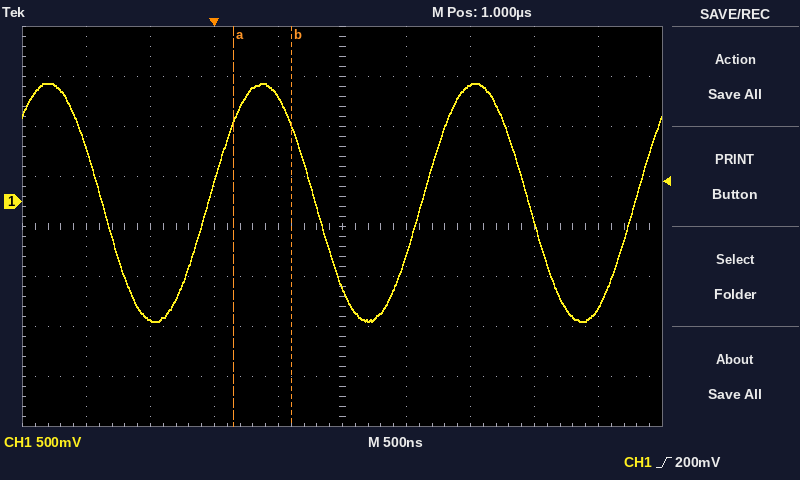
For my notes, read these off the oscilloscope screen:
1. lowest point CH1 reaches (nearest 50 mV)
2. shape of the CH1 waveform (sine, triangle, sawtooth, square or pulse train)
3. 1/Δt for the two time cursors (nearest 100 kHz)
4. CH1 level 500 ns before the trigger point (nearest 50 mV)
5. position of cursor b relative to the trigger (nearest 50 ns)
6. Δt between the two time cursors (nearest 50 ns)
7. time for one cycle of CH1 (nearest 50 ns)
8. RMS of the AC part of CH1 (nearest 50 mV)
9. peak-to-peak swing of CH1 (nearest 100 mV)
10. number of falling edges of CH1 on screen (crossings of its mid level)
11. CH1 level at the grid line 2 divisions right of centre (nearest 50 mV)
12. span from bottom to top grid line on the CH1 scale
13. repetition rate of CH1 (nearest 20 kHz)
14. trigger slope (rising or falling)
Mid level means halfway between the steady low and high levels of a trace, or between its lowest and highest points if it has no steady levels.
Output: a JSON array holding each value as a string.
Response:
["-1.20 V", "sine", "2.2 MHz", "-1.20 V", "+600 ns", "450 ns", "1.65 µs", "850 mV", "2.40 V", "3", "1.15 V", "4 V", "600 kHz", "rising"]
